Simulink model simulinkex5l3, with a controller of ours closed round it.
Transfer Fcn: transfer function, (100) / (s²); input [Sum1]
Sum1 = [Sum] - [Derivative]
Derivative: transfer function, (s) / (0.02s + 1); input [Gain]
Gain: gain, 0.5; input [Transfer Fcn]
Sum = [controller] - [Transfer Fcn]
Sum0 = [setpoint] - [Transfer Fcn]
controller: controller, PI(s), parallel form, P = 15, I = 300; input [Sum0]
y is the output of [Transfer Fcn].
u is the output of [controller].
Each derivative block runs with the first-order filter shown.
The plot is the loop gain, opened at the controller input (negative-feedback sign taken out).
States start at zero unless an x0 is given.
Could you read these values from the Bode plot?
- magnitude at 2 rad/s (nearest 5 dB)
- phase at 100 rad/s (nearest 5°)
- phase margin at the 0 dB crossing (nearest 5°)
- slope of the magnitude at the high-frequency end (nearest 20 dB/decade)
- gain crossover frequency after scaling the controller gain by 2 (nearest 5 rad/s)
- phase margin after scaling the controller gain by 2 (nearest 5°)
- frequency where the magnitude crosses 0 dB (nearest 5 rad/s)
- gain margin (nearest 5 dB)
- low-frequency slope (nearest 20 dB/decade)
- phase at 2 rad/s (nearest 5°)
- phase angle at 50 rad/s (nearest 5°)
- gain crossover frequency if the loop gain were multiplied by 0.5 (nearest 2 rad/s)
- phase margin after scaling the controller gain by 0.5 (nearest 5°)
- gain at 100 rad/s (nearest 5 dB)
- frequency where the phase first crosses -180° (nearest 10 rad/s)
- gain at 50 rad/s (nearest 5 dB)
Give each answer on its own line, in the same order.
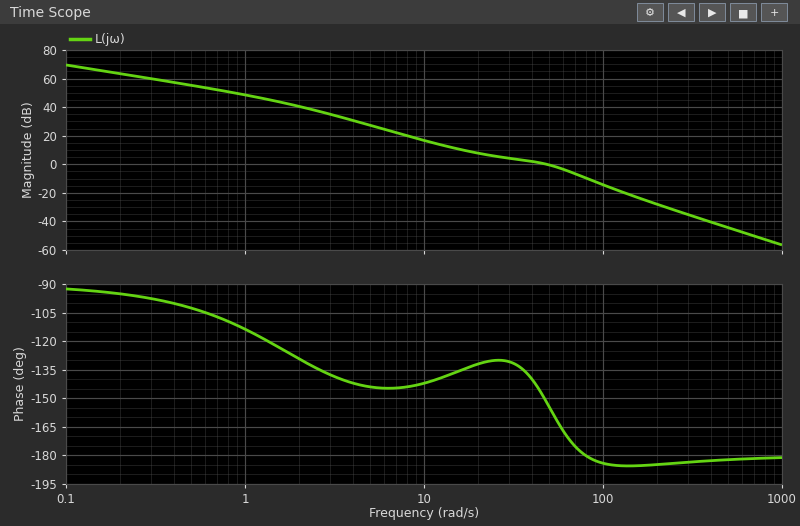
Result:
40 dB
-185°
30°
-40 dB/decade
70 rad/s
5°
50 rad/s
10 dB
-20 dB/decade
-130°
-155°
24 rad/s
50°
-15 dB
80 rad/s
0 dB
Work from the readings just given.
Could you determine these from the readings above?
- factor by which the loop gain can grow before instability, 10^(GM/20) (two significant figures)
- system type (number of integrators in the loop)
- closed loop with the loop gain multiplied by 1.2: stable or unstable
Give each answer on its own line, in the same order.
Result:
3.2
1
stable
